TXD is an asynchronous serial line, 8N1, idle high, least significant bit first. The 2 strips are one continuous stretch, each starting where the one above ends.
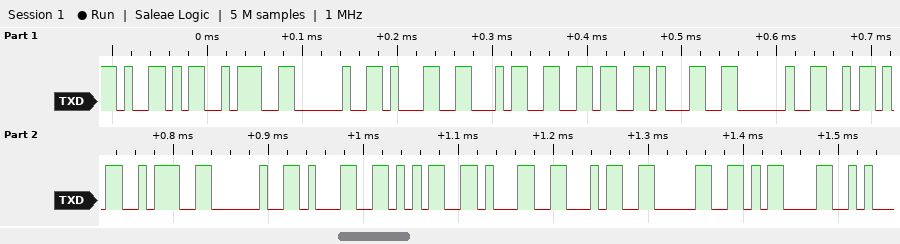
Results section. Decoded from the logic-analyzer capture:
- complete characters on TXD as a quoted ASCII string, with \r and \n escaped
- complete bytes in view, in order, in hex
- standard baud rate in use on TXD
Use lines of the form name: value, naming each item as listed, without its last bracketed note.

complete characters on TXD as a quoted ASCII string, with \r and \n escaped: "Y: 1461 Z: 15140\r"
complete bytes in view, in order, in hex: 59 3A 20 31 34 36 31 20 5A 3A 20 31 35 31 34 30 0D
standard baud rate in use on TXD: 115200 baud
